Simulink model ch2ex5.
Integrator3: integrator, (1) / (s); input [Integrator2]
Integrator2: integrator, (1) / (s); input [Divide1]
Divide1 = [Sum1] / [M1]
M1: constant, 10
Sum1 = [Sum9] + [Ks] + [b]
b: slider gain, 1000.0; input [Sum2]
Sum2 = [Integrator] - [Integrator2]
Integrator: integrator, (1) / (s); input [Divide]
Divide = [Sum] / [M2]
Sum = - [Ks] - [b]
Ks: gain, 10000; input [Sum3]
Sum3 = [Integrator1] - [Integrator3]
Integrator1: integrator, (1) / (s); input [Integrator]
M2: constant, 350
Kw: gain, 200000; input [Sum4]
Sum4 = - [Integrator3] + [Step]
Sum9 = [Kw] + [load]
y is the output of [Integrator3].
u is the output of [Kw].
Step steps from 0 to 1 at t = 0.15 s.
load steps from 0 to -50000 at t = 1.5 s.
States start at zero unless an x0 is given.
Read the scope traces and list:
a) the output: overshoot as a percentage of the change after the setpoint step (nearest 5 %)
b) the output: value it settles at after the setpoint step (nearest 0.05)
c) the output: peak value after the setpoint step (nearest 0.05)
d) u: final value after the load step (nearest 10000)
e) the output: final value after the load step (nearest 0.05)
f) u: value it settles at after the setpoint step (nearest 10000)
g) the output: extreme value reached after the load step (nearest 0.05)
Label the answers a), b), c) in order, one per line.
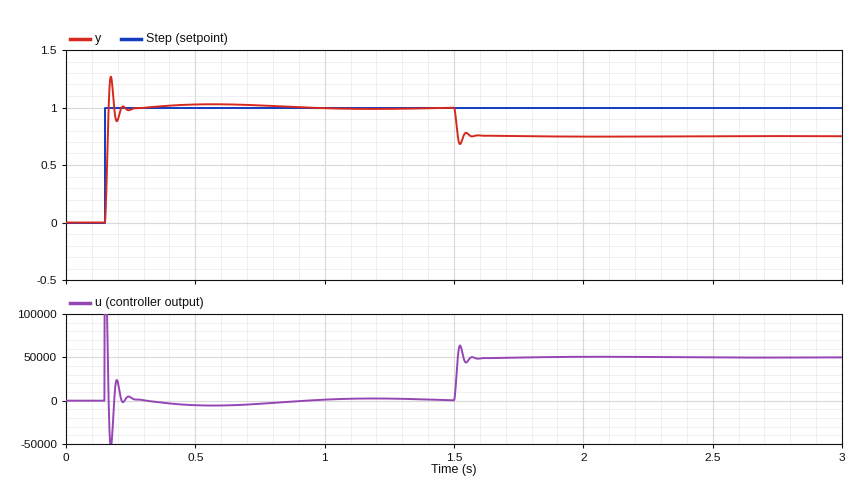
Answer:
a) 25 %
b) 1.00
c) 1.25
d) 50000
e) 0.75
f) 0
g) 0.70
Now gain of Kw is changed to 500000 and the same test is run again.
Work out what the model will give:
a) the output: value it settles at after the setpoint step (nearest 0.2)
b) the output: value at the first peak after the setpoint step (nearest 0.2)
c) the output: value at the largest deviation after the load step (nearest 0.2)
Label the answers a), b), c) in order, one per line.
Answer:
a) 1.0
b) 1.4
c) 0.8
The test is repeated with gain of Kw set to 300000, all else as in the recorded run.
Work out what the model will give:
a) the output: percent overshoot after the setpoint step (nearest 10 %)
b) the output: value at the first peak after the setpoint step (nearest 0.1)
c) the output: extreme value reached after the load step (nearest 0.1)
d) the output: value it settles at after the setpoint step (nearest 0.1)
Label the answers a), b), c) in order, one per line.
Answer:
a) 40 %
b) 1.4
c) 0.8
d) 1.0
